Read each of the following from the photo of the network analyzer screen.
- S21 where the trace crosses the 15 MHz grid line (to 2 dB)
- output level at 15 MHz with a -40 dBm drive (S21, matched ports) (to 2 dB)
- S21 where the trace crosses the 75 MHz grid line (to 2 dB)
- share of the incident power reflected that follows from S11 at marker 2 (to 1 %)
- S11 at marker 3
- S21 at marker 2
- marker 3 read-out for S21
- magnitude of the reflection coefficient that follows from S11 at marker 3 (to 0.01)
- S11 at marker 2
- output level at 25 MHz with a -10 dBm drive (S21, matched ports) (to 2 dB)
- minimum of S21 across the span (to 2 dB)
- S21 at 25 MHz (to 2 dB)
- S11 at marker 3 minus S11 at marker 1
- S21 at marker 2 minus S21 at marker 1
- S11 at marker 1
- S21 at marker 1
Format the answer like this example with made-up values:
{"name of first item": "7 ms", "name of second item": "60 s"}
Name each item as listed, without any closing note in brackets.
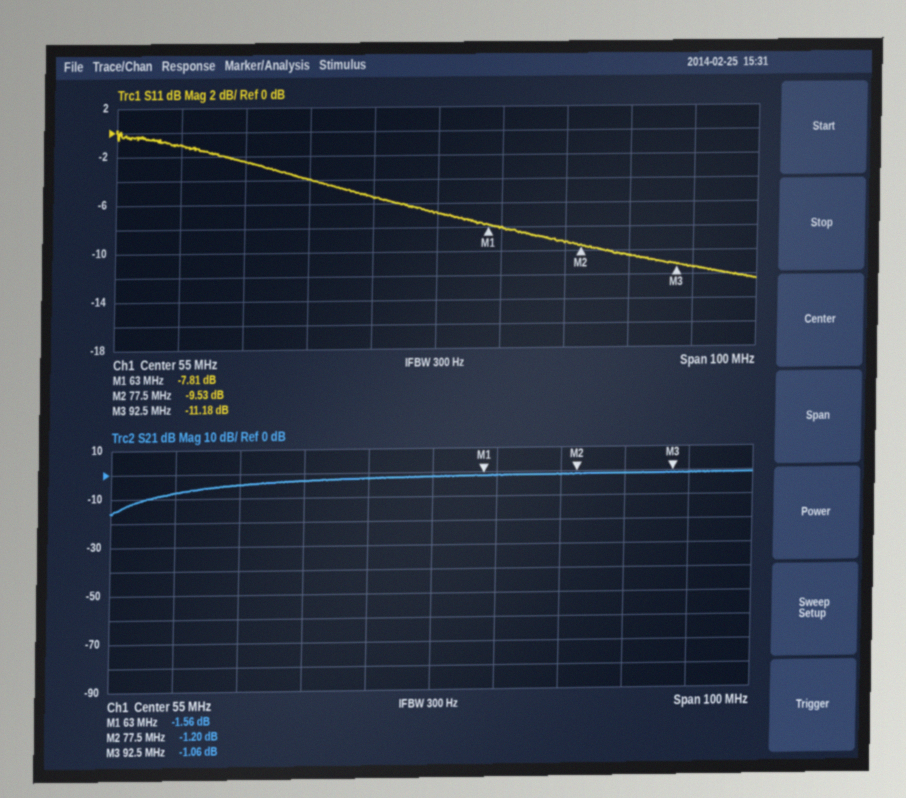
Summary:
{"S21 where the trace crosses the 15 MHz grid line": "-8 dB", "output level at 15 MHz with a -40 dBm drive (S21, matched ports)": "-48 dBm", "S21 where the trace crosses the 75 MHz grid line": "-2 dB", "share of the incident power reflected that follows from S11 at marker 2": "11 %", "S11 at marker 3": "-11.18 dB", "S21 at marker 2": "-1.20 dB", "marker 3 read-out for S21": "-1.06 dB", "magnitude of the reflection coefficient that follows from S11 at marker 3": "0.28", "S11 at marker 2": "-9.53 dB", "output level at 25 MHz with a -10 dBm drive (S21, matched ports)": "-14 dBm", "minimum of S21 across the span": "-16 dB", "S21 at 25 MHz": "-4 dB", "S11 at marker 3 minus S11 at marker 1": "-3.37 dB", "S21 at marker 2 minus S21 at marker 1": "0.36 dB", "S11 at marker 1": "-7.81 dB", "S21 at marker 1": "-1.56 dB"}
